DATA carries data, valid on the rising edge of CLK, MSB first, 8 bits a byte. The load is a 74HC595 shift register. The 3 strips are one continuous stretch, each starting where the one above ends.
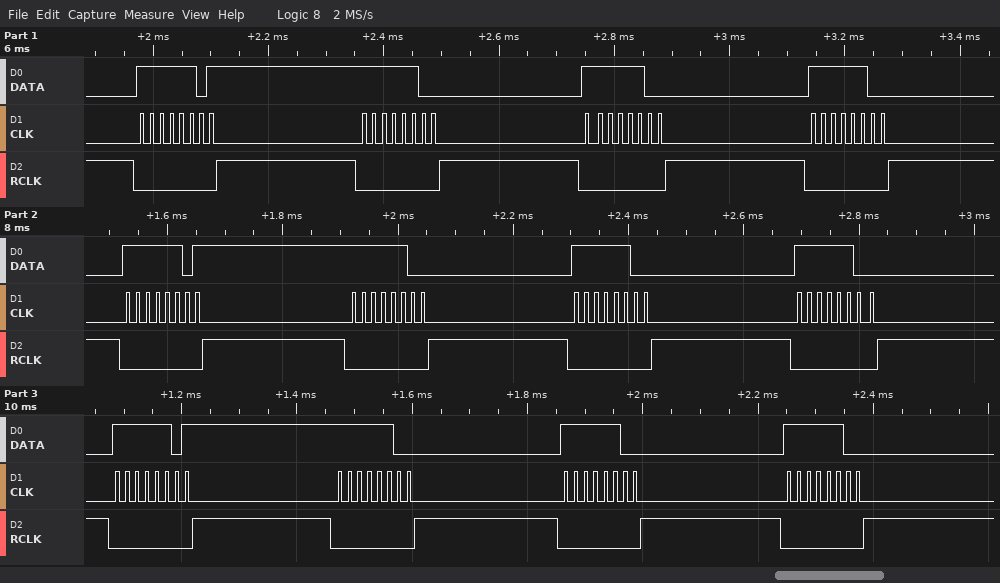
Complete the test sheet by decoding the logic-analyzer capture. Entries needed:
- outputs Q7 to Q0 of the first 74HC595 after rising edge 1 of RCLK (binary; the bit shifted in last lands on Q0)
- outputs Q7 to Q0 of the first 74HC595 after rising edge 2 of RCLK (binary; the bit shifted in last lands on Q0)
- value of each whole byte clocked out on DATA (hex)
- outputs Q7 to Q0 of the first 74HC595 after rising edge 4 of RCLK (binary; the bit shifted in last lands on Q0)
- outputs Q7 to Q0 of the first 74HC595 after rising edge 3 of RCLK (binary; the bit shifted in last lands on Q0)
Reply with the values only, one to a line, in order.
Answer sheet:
11111101
11111100
FD FC FC FC FD FC FC FC FD FC FC FC
11111100
11111100
